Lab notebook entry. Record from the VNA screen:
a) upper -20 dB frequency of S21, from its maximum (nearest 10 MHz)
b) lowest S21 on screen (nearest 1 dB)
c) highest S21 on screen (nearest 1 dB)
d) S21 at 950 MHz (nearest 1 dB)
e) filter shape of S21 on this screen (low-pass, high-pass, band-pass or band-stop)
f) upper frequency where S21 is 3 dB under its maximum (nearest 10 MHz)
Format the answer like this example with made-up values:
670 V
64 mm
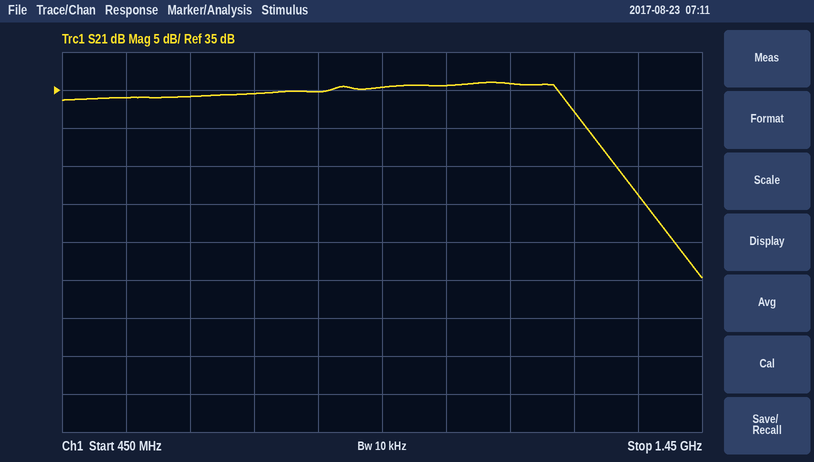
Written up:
1.40 GHz
10 dB
36 dB
35 dB
low-pass
1.24 GHz
